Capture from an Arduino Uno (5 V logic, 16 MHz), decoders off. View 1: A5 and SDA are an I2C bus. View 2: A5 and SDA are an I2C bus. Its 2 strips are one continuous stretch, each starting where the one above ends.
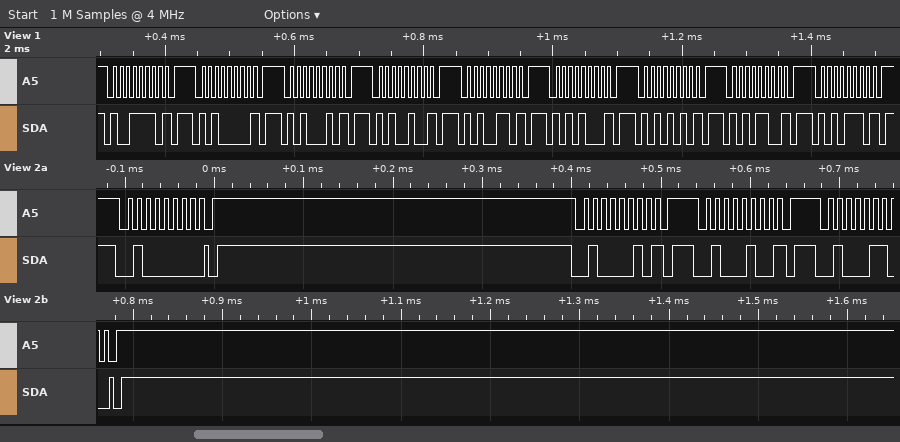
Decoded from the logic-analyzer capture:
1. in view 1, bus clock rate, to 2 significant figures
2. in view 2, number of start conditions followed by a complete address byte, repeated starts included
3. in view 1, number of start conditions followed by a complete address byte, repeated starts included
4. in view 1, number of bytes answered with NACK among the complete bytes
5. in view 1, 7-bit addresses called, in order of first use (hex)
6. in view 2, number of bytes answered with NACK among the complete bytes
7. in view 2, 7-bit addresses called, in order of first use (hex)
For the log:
100 kHz
4
9
9
0x4F 0x50 0x51 0x52 0x53 0x54 0x55 0x56 0x57
2
0x20 0x21 0x22 0x23
